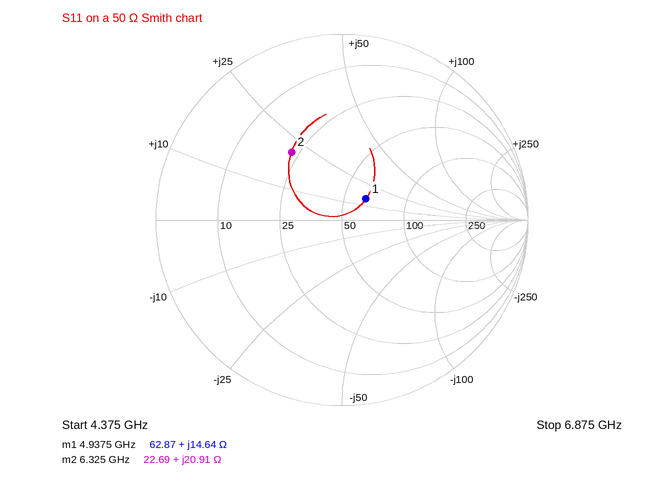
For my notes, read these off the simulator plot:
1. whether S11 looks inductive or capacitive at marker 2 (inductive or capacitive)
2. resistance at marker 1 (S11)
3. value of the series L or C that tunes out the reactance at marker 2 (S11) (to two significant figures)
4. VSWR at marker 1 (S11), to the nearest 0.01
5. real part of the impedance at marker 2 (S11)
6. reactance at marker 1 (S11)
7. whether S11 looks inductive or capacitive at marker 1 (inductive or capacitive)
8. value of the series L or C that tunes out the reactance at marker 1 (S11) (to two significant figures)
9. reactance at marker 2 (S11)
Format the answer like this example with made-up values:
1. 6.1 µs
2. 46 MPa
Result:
1. inductive
2. 62.87 Ω
3. 1.2 pF
4. 1.41
5. 22.69 Ω
6. +14.64 Ω
7. inductive
8. 2.2 pF
9. +20.91 Ω
